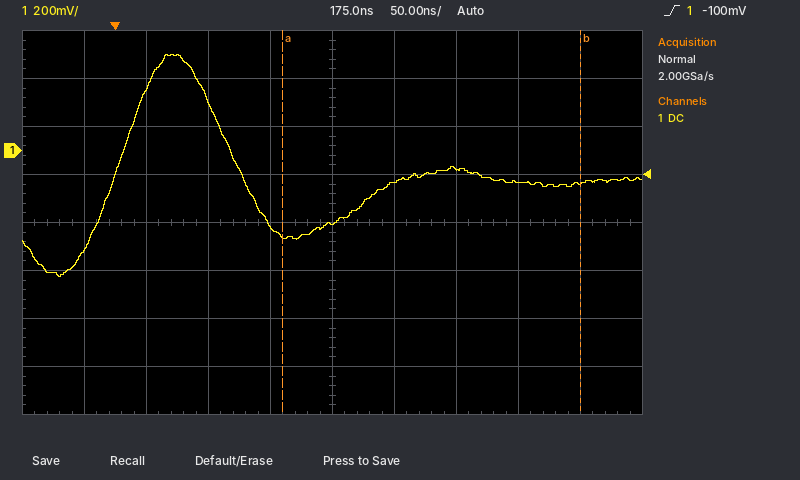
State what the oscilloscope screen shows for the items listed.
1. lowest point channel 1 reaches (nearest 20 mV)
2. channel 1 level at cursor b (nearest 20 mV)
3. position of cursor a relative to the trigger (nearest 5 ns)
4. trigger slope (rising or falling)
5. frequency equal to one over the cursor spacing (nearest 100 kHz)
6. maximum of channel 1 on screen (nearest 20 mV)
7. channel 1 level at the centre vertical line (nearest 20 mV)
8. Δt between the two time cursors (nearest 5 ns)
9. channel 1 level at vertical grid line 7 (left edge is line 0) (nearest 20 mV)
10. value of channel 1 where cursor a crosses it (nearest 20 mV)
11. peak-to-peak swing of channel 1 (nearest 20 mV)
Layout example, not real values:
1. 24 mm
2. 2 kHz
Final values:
1. -520 mV
2. -140 mV
3. +135 ns
4. rising
5. 4.2 MHz
6. 400 mV
7. -300 mV
8. 240 ns
9. -80 mV
10. -360 mV
11. 920 mV
